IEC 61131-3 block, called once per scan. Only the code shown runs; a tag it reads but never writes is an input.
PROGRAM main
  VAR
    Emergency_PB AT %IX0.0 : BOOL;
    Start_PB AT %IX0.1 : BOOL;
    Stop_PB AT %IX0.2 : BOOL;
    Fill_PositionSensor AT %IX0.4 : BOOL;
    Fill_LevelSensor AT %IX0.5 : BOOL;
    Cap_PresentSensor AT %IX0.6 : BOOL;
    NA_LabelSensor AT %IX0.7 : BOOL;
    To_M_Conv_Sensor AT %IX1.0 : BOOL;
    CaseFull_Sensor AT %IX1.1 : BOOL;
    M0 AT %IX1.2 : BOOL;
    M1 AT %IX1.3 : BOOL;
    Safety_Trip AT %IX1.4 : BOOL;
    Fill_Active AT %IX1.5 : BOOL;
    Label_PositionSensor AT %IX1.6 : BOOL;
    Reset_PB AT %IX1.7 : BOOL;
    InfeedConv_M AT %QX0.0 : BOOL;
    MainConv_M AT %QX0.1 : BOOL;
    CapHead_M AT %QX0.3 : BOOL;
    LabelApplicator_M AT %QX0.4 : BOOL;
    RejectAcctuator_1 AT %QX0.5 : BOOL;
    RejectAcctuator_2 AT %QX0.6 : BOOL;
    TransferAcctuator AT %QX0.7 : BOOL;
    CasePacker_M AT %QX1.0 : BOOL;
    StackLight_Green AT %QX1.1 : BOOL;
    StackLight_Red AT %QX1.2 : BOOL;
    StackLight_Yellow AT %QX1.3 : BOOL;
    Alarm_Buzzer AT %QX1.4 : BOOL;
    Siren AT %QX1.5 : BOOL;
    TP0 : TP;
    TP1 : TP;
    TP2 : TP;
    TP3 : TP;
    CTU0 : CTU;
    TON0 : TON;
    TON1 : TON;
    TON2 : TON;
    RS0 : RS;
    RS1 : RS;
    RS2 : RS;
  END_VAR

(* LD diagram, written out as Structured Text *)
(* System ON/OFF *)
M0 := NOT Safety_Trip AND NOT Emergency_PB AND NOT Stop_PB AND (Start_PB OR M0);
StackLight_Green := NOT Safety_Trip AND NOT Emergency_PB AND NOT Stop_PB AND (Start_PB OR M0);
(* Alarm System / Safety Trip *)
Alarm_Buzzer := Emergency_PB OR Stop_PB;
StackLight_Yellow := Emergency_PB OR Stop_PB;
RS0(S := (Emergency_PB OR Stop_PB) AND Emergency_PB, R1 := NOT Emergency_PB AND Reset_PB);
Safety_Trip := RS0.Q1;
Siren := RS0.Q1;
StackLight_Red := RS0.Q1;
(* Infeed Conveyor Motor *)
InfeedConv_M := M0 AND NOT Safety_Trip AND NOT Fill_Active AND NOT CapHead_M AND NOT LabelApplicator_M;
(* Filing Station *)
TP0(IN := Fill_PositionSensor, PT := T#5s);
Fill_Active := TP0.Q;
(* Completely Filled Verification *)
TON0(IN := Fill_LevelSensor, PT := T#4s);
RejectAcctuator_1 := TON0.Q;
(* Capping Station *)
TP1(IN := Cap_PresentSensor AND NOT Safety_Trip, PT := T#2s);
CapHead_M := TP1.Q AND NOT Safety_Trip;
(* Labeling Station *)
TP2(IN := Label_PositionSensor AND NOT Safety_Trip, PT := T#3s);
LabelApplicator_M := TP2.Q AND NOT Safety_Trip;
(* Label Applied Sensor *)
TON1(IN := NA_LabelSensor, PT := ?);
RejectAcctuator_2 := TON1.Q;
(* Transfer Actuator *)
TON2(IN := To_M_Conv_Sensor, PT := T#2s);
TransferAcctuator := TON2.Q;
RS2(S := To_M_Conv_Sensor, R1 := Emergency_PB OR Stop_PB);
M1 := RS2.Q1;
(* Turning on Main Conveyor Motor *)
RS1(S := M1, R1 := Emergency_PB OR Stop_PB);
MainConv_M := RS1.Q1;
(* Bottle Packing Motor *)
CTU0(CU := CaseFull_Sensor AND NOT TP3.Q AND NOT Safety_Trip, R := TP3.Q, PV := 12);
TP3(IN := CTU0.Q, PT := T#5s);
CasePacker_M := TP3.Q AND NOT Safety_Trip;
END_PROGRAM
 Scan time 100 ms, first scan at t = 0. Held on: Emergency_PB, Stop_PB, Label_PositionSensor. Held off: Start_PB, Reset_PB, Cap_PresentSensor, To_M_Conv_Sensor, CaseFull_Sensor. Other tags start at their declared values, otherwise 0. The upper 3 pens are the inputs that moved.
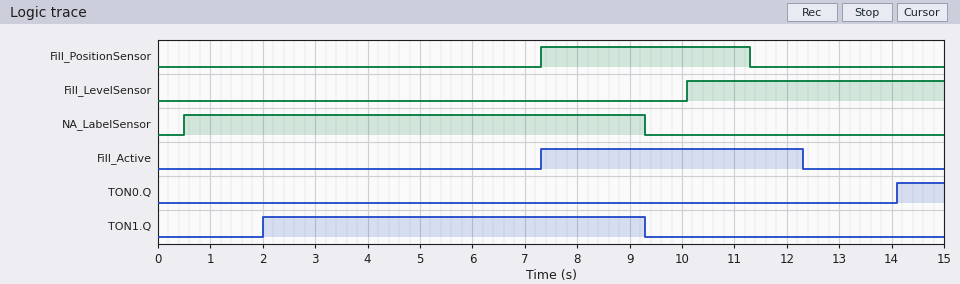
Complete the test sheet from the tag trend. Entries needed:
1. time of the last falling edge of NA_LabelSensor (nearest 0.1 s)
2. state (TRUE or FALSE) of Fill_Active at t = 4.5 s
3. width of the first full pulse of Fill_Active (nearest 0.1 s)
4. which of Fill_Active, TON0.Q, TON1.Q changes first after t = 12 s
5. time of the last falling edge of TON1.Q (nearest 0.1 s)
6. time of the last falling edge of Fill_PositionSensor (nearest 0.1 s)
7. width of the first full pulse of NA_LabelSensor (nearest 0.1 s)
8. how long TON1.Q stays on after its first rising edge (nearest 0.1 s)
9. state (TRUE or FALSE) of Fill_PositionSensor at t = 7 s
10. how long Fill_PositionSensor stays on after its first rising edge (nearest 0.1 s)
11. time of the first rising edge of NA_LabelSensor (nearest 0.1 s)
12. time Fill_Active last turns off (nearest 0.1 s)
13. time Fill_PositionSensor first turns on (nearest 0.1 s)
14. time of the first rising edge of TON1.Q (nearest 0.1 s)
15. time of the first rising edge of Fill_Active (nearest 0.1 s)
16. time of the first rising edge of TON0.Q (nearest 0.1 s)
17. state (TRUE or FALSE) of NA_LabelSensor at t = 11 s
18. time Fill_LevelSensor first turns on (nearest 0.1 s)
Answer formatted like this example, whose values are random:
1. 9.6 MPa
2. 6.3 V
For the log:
1. 9.3 s
2. FALSE
3. 5.0 s
4. Fill_Active
5. 9.3 s
6. 11.3 s
7. 8.8 s
8. 7.3 s
9. FALSE
10. 4.0 s
11. 0.5 s
12. 12.3 s
13. 7.3 s
14. 2.0 s
15. 7.3 s
16. 14.1 s
17. FALSE
18. 10.1 s
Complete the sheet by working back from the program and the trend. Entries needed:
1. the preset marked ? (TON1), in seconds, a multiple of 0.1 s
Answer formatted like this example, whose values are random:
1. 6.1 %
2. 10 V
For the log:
1. 1.5 s
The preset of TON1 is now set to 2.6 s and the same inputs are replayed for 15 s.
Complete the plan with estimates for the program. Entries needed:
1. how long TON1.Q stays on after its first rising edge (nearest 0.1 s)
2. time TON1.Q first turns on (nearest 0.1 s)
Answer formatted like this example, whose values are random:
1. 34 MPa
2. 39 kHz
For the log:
1. 6.2 s
2. 3.1 s
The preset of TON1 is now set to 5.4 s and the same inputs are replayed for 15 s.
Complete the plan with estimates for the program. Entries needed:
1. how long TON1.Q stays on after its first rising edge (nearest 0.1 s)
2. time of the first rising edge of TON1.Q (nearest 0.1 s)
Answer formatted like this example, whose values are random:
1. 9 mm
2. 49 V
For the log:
1. 3.4 s
2. 5.9 s
